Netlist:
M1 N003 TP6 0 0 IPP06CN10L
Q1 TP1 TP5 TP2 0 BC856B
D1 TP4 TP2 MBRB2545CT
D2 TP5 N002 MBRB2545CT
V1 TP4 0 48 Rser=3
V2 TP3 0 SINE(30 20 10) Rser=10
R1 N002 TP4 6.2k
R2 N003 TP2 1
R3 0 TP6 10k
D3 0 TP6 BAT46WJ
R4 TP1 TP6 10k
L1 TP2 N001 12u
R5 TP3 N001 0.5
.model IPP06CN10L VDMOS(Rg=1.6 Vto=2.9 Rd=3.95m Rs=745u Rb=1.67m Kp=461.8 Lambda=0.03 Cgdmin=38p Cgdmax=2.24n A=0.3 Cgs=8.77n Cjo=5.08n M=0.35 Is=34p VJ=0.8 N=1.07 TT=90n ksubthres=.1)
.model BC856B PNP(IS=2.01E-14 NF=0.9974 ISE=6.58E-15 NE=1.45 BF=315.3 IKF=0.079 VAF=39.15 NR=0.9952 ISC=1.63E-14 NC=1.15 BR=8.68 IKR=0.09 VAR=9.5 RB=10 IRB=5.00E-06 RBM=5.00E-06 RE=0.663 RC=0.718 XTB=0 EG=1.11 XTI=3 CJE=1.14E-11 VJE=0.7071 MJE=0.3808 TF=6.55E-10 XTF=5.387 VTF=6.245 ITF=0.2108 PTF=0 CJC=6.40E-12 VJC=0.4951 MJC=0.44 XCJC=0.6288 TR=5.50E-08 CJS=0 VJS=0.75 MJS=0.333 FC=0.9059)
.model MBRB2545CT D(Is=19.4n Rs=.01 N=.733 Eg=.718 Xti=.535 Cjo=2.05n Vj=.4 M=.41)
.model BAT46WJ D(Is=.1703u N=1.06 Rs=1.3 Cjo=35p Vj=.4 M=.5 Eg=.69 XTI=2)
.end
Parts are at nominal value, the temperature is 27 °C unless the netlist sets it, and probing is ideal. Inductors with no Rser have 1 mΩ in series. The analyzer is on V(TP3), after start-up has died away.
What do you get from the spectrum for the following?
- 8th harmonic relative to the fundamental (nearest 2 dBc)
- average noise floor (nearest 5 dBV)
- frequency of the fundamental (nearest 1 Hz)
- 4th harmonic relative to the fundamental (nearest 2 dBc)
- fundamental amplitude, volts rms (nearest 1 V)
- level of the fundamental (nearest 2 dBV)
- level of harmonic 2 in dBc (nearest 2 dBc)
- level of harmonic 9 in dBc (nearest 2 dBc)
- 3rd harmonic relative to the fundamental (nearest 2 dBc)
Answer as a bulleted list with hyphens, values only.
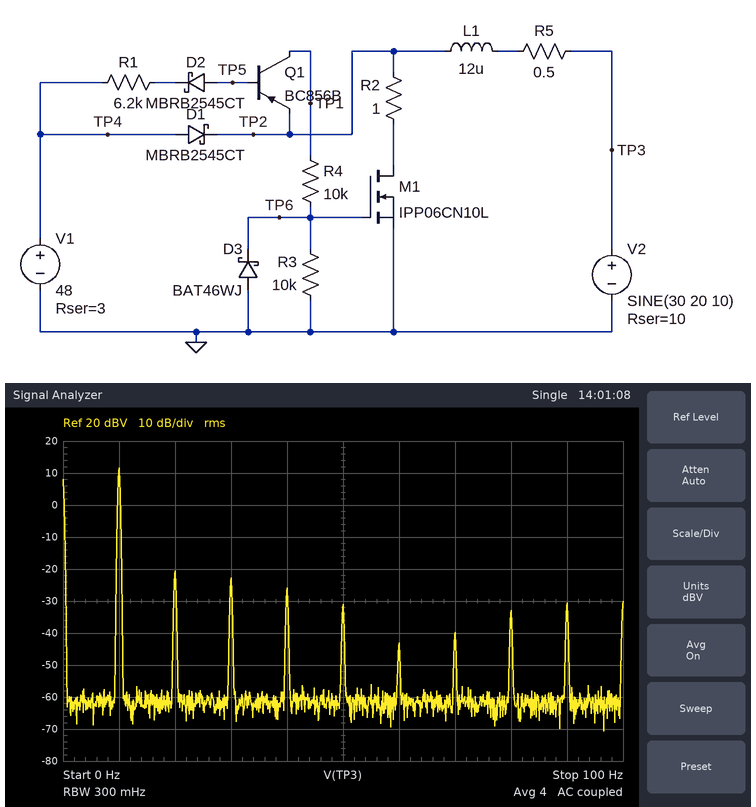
- -44 dBc
- -60 dBV
- 10 Hz
- -38 dBc
- 4 V
- 12 dBV
- -32 dBc
- -42 dBc
- -34 dBc
